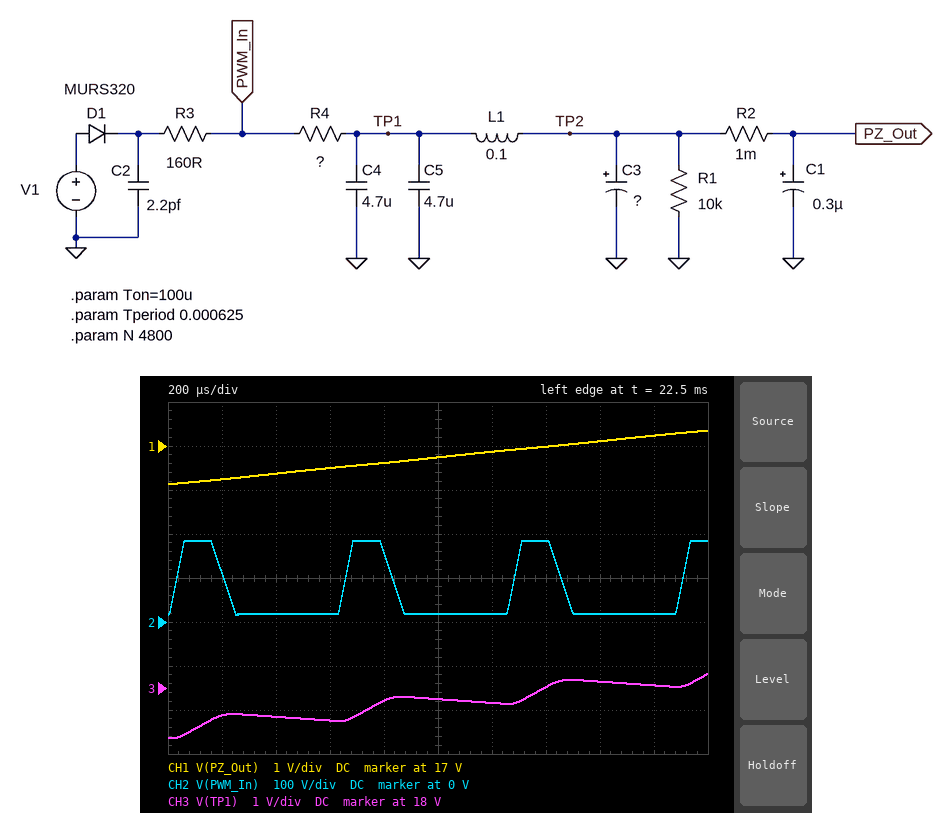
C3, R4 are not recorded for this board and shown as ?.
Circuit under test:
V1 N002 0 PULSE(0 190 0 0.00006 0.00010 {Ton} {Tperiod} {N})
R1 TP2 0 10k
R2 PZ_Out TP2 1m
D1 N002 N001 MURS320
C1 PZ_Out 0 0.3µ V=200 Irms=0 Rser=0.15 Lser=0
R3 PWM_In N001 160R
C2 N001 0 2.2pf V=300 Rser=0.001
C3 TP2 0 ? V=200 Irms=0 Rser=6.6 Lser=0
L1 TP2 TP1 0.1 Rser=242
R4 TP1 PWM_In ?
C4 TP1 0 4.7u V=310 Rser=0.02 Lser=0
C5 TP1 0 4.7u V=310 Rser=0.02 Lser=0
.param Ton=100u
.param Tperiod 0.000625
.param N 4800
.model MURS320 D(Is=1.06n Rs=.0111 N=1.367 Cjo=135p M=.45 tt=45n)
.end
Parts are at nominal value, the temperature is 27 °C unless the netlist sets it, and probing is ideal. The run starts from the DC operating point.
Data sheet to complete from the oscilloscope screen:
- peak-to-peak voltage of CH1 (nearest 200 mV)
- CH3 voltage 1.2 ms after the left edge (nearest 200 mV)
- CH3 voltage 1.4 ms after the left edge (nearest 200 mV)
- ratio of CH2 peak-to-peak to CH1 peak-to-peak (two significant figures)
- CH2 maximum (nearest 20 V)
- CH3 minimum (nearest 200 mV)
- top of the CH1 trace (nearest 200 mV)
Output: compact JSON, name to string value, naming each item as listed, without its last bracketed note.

{"peak-to-peak voltage of CH1": "1.2 V", "CH3 voltage 1.2 ms after the left edge": "17.6 V", "CH3 voltage 1.4 ms after the left edge": "18.0 V", "ratio of CH2 peak-to-peak to CH1 peak-to-peak": "140", "CH2 maximum": "180 V", "CH3 minimum": "16.8 V", "top of the CH1 trace": "17.4 V"}
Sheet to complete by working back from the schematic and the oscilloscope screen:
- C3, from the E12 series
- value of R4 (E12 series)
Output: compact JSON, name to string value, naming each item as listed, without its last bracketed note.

{"C3, from the E12 series": "3.3 µF", "value of R4": "4.7 kΩ"}
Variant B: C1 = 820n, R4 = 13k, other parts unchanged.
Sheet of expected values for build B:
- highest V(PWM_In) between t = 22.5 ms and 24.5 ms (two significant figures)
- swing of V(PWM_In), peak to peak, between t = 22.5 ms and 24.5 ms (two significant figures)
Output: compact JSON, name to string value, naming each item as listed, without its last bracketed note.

{"highest V(PWM_In) between t = 22.5 ms and 24.5 ms": "190 V", "swing of V(PWM_In), peak to peak, between t = 22.5 ms and 24.5 ms": "180 V"}
